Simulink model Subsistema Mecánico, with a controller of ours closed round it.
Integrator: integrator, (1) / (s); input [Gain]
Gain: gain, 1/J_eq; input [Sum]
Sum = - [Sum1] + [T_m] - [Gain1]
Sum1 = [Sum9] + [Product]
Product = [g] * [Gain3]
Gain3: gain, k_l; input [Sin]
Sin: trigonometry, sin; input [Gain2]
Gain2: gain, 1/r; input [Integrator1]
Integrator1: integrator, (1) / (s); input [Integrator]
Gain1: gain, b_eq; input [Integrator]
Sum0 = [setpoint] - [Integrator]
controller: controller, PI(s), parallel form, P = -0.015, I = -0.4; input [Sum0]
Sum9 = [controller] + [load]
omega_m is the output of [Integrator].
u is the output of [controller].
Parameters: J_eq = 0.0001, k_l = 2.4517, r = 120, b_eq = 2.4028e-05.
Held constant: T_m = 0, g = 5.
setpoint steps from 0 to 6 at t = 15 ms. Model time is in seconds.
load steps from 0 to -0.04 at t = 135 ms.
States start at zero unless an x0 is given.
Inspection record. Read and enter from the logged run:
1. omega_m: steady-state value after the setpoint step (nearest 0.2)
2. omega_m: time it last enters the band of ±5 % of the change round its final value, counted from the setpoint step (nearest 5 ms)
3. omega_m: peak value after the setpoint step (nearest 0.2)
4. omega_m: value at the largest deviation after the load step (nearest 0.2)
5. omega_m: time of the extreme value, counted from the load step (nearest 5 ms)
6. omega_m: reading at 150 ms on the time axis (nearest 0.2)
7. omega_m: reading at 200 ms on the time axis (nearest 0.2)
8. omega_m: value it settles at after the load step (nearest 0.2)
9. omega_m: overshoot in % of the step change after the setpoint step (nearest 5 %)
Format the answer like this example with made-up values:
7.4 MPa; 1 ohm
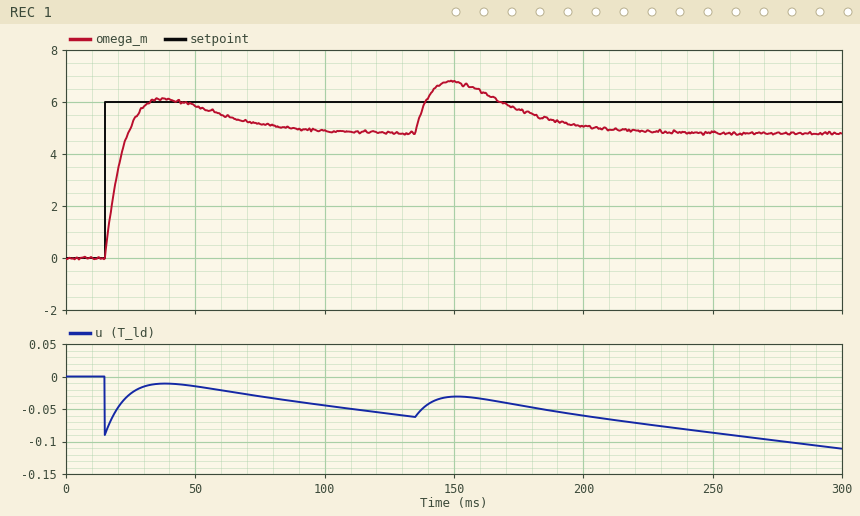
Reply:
4.8; 70 ms; 6.2; 6.8; 15 ms; 6.8; 5.0; 4.8; 30 %
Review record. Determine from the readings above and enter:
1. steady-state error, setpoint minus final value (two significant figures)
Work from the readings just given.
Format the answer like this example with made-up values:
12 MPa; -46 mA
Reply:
1.2
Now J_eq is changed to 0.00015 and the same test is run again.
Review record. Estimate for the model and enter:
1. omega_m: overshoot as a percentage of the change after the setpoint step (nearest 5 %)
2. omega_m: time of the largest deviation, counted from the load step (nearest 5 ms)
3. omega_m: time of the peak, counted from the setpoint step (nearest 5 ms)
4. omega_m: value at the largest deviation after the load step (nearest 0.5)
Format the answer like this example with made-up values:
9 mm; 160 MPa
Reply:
30 %; 20 ms; 30 ms; 6.5
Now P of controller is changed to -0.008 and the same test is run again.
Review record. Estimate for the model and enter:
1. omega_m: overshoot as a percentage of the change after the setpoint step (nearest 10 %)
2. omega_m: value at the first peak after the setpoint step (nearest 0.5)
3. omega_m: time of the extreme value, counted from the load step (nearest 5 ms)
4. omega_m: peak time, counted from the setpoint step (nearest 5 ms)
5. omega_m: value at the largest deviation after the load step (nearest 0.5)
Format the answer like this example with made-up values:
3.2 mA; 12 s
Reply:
40 %; 6.5; 15 ms; 30 ms; 7.5
